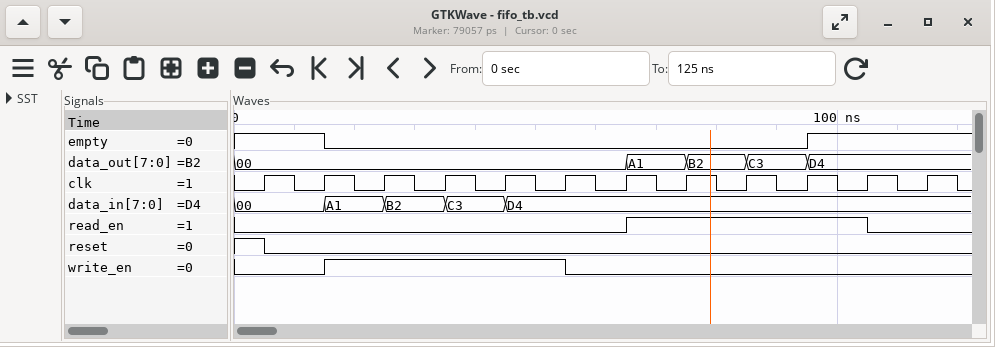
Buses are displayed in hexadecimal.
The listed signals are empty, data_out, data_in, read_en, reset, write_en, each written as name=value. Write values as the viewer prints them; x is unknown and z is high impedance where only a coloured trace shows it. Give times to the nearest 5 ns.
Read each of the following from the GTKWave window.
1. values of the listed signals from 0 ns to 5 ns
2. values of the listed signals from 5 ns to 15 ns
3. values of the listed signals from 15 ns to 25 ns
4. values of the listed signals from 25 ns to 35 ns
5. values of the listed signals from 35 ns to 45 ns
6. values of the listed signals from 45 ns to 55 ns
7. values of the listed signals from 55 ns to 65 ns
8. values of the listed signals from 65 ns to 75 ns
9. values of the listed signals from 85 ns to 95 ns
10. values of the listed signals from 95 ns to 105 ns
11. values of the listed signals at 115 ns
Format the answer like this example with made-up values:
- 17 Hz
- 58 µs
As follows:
- empty=1, data_out=00, data_in=00, read_en=0, reset=1, write_en=0
- empty=1, data_out=00, data_in=00, read_en=0, reset=0, write_en=0
- empty=0, data_out=00, data_in=A1, read_en=0, reset=0, write_en=1
- empty=0, data_out=00, data_in=B2, read_en=0, reset=0, write_en=1
- empty=0, data_out=00, data_in=C3, read_en=0, reset=0, write_en=1
- empty=0, data_out=00, data_in=D4, read_en=0, reset=0, write_en=1
- empty=0, data_out=00, data_in=D4, read_en=0, reset=0, write_en=0
- empty=0, data_out=A1, data_in=D4, read_en=1, reset=0, write_en=0
- empty=0, data_out=C3, data_in=D4, read_en=1, reset=0, write_en=0
- empty=1, data_out=D4, data_in=D4, read_en=1, reset=0, write_en=0
- empty=1, data_out=D4, data_in=D4, read_en=0, reset=0, write_en=0
